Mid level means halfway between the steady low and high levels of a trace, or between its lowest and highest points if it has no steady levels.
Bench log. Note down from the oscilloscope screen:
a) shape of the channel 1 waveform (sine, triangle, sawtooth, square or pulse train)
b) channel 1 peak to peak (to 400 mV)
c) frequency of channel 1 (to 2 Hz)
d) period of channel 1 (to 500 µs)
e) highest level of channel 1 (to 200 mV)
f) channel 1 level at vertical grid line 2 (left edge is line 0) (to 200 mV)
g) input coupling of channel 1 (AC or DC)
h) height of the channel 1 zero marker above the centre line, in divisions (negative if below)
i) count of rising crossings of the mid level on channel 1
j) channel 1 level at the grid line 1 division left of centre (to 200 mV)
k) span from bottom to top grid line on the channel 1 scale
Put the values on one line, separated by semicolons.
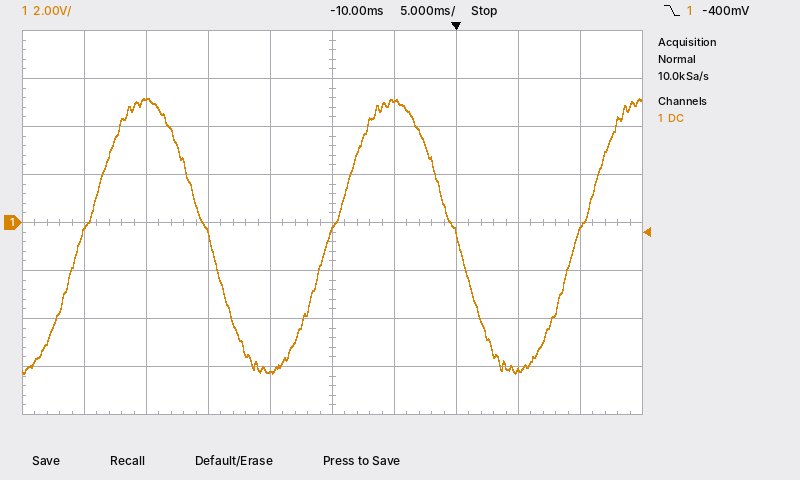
sine; 11.6 V; 50 Hz; 20.0 ms; 5.2 V; 5.2 V; DC; 0.0 div; 3; -6.2 V; 16 V
